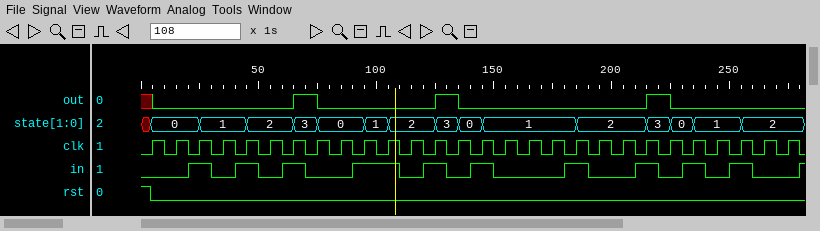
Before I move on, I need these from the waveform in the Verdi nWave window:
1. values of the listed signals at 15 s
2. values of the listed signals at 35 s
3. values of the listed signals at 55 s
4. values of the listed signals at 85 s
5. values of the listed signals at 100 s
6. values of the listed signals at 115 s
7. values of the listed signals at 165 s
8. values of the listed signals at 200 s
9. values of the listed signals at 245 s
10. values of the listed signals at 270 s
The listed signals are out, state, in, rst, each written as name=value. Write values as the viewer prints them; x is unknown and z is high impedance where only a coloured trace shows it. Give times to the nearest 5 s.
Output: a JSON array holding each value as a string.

["out=0, state=0, in=0, rst=0", "out=0, state=1, in=0, rst=0", "out=0, state=2, in=0, rst=0", "out=0, state=0, in=0, rst=0", "out=0, state=1, in=1, rst=0", "out=0, state=2, in=0, rst=0", "out=0, state=1, in=0, rst=0", "out=0, state=2, in=0, rst=0", "out=0, state=1, in=0, rst=0", "out=0, state=2, in=0, rst=0"]
